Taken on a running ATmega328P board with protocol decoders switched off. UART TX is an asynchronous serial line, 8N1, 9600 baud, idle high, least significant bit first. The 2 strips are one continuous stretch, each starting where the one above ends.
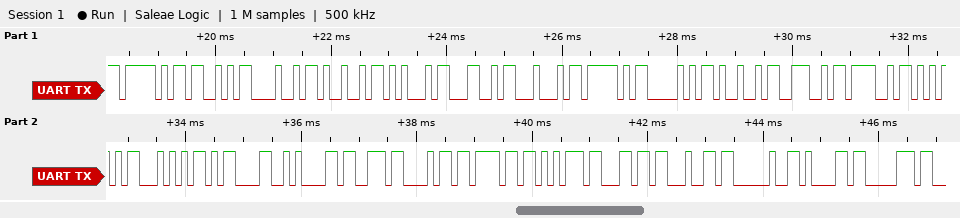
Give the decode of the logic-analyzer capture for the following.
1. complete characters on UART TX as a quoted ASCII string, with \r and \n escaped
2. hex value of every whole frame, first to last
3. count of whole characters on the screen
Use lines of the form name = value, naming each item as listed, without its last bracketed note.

complete characters on UART TX as a quoted ASCII string, with \r and \n escaped = "_SHIELD_PINOUT\r\nshould ap"
hex value of every whole frame, first to last = 5F 53 48 49 45 4C 44 5F 50 49 4E 4F 55 54 0D 0A 73 68 6F 75 6C 64 20 61 70
count of whole characters on the screen = 25
